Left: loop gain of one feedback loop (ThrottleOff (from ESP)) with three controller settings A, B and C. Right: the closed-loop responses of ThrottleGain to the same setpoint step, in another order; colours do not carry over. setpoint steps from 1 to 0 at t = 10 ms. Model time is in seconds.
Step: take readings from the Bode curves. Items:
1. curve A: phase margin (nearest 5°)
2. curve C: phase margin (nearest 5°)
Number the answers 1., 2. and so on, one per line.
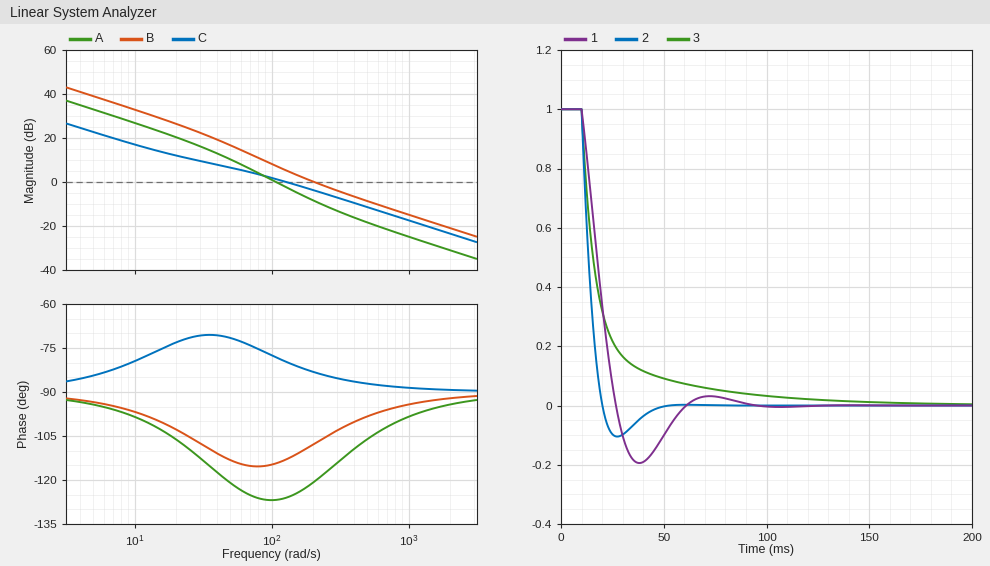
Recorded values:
1. 55°
2. 100°
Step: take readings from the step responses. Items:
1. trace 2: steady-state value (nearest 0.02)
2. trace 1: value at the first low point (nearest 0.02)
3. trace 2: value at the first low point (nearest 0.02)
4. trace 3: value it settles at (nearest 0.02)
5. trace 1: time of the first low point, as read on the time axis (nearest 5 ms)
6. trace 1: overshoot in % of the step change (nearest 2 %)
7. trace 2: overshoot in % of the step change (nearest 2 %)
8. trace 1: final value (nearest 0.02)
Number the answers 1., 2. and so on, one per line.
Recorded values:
1. 0.00
2. -0.20
3. -0.10
4. 0.00
5. 40 ms
6. 20 %
7. 10 %
8. 0.00
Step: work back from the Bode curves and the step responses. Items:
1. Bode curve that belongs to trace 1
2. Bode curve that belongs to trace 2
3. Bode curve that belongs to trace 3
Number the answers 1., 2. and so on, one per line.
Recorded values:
1. A
2. B
3. C
